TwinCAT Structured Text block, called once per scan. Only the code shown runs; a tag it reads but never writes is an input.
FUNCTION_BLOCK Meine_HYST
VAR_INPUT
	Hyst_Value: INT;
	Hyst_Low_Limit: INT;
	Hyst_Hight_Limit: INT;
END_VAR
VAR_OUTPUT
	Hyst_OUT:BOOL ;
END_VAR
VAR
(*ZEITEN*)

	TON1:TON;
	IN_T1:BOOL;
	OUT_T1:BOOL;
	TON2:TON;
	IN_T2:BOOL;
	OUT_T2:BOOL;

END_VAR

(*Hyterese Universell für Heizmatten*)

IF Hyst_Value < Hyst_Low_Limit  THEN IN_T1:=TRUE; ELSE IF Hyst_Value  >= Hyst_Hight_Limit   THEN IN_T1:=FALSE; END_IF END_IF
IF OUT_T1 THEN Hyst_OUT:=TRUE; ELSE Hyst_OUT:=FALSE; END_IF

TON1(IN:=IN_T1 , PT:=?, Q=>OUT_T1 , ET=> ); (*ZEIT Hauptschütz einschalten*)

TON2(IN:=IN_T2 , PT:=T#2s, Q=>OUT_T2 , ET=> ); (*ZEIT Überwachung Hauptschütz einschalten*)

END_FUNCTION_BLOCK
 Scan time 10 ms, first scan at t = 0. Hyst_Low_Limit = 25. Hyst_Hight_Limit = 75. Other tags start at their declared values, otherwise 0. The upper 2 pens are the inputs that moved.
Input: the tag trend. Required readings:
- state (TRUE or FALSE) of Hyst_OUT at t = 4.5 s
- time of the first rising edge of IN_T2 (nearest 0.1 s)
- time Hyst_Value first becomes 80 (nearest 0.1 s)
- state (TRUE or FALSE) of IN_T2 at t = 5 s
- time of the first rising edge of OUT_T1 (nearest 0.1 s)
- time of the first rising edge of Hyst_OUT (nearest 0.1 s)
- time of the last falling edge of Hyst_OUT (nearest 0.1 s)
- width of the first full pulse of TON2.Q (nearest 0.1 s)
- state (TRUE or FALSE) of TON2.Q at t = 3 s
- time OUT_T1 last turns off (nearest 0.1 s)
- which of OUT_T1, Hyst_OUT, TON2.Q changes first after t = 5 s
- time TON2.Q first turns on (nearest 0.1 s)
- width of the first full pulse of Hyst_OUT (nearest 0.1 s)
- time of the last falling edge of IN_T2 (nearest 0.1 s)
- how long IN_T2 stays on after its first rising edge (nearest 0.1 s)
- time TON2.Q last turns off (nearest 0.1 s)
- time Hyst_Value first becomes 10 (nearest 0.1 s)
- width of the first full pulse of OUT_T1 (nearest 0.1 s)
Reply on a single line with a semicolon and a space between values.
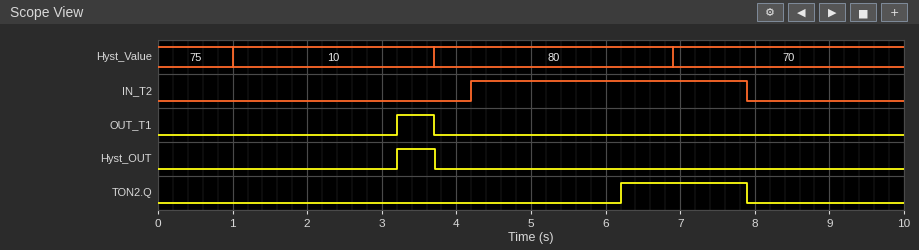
FALSE; 4.2 s; 3.7 s; TRUE; 3.2 s; 3.2 s; 3.7 s; 1.7 s; FALSE; 3.7 s; TON2.Q; 6.2 s; 0.5 s; 7.9 s; 3.7 s; 7.9 s; 1.0 s; 0.5 s
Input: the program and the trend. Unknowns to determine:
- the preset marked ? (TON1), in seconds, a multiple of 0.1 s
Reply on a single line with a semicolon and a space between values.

2.2 s
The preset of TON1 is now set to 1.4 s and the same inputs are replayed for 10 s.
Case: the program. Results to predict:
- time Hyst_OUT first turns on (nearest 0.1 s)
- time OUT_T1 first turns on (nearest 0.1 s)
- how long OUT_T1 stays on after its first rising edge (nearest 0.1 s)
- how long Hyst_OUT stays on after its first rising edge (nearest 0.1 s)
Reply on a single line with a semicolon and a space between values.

2.4 s; 2.4 s; 1.3 s; 1.3 s
